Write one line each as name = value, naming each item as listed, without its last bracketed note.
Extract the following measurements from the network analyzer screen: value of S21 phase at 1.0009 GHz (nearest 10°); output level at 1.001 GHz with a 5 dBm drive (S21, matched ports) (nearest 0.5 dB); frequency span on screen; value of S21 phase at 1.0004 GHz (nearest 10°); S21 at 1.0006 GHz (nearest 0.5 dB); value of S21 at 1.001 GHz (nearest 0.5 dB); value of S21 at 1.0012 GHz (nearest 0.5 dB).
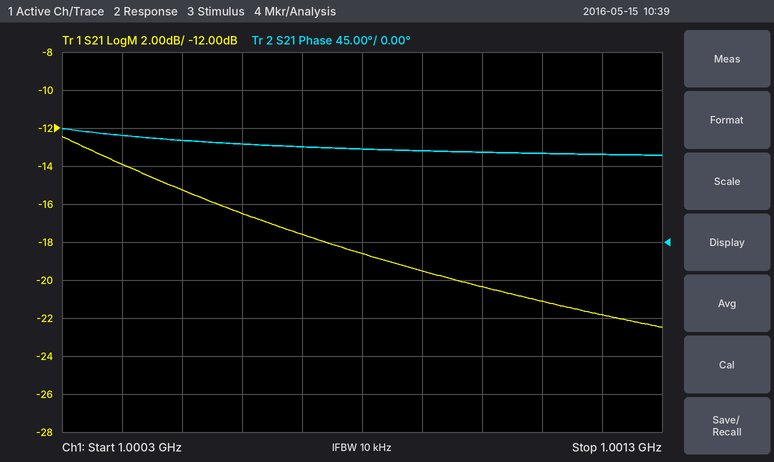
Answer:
value of S21 phase at 1.0009 GHz = 110°
output level at 1.001 GHz with a 5 dBm drive (S21, matched ports) = -15.5 dBm
frequency span on screen = 1 MHz
value of S21 phase at 1.0004 GHz = 130°
S21 at 1.0006 GHz = -16.5 dB
value of S21 at 1.001 GHz = -20.5 dB
value of S21 at 1.0012 GHz = -22.0 dB
